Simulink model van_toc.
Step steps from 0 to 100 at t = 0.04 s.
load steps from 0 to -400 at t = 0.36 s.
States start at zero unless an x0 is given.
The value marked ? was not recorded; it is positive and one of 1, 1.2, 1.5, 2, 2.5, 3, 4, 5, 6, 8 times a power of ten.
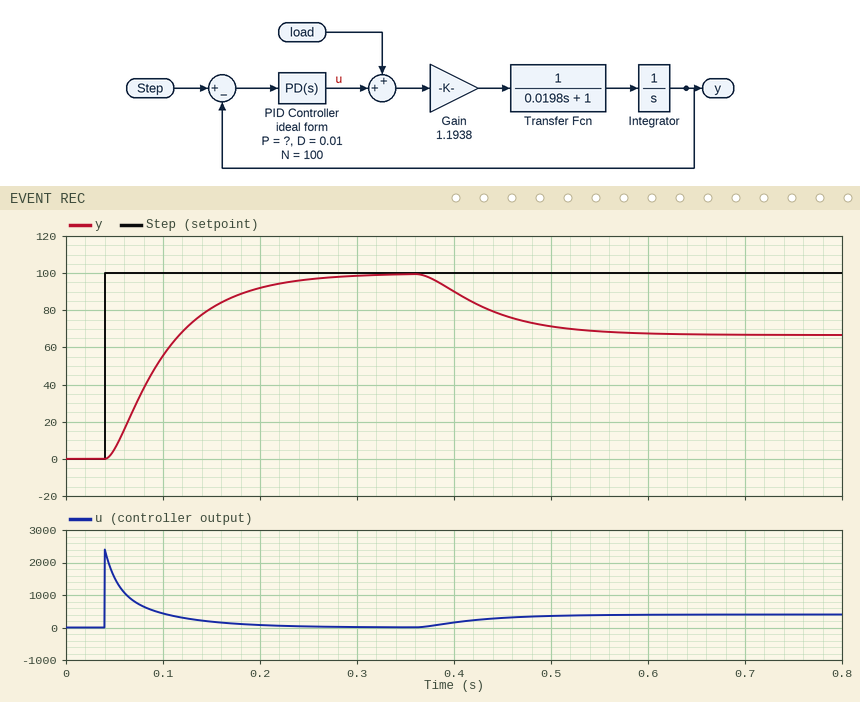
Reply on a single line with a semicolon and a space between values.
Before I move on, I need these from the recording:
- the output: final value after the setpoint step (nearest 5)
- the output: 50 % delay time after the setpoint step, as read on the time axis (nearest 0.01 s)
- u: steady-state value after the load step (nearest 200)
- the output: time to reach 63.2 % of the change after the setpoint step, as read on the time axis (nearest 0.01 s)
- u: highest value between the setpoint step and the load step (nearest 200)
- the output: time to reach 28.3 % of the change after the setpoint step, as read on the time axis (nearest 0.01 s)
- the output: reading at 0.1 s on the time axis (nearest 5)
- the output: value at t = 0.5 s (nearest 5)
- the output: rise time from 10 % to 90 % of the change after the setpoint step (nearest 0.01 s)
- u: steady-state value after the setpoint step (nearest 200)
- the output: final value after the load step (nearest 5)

100; 0.09 s; 400; 0.11 s; 2400; 0.07 s; 55; 70; 0.13 s; 0; 65
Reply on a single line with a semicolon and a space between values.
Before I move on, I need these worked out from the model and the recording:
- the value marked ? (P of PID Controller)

12
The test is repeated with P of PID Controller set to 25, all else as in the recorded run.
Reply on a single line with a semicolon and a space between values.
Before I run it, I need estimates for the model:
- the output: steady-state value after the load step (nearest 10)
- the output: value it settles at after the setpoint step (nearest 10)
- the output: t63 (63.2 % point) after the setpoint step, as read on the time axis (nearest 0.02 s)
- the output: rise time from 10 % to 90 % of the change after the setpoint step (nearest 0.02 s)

80; 100; 0.08 s; 0.06 s
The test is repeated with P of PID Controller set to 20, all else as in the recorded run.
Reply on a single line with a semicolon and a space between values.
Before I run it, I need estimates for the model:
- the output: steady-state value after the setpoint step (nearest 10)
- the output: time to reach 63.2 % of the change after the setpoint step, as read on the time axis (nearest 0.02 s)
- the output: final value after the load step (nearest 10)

100; 0.08 s; 80
